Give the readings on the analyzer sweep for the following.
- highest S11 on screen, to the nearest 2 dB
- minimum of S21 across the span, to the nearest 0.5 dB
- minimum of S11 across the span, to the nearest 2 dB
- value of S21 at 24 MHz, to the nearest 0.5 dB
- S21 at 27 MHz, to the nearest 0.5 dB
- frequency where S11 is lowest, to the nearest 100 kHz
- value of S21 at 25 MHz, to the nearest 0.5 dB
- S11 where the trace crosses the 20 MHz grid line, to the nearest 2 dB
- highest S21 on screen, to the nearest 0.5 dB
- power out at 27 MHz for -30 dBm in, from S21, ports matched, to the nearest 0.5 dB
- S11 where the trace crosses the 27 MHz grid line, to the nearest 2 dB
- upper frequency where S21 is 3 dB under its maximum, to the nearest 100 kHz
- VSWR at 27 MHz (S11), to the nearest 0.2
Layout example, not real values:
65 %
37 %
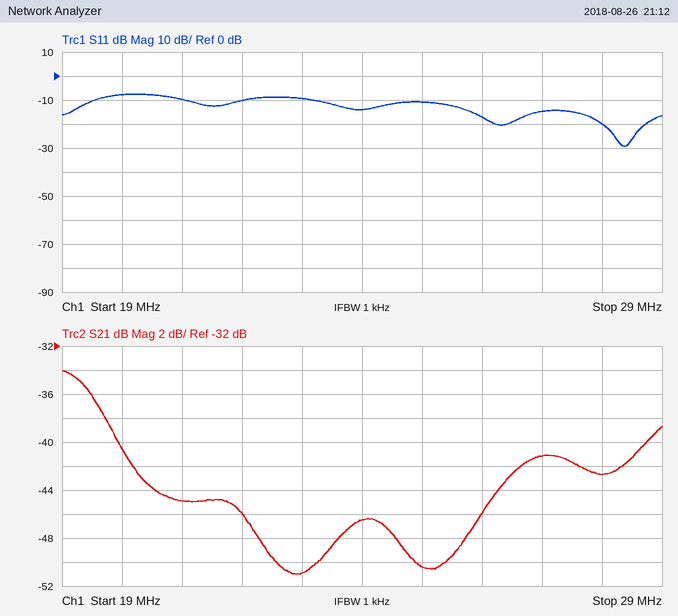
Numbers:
-8 dB
-51.0 dB
-30 dB
-46.5 dB
-41.0 dB
28.4 MHz
-50.5 dB
-8 dB
-34.0 dB
-71.0 dBm
-14 dB
19.6 MHz
1.4
